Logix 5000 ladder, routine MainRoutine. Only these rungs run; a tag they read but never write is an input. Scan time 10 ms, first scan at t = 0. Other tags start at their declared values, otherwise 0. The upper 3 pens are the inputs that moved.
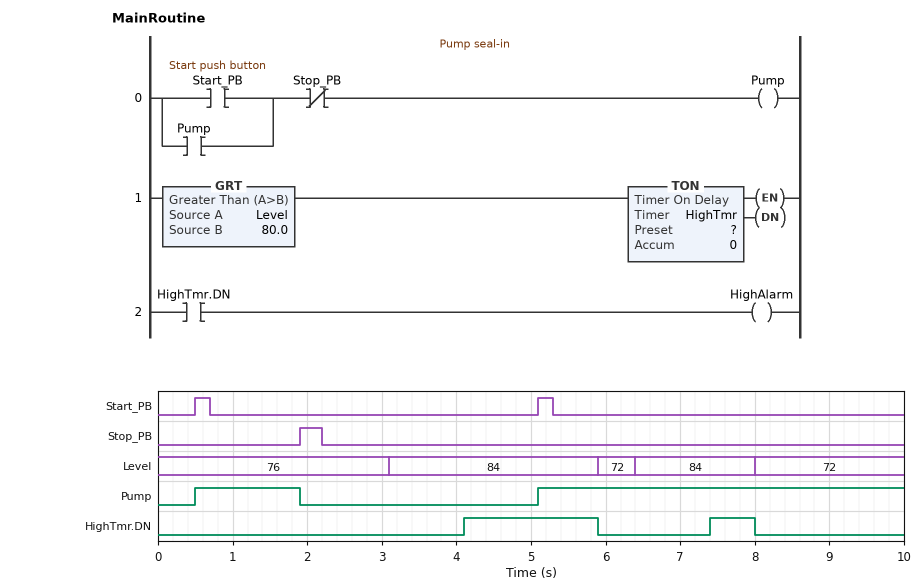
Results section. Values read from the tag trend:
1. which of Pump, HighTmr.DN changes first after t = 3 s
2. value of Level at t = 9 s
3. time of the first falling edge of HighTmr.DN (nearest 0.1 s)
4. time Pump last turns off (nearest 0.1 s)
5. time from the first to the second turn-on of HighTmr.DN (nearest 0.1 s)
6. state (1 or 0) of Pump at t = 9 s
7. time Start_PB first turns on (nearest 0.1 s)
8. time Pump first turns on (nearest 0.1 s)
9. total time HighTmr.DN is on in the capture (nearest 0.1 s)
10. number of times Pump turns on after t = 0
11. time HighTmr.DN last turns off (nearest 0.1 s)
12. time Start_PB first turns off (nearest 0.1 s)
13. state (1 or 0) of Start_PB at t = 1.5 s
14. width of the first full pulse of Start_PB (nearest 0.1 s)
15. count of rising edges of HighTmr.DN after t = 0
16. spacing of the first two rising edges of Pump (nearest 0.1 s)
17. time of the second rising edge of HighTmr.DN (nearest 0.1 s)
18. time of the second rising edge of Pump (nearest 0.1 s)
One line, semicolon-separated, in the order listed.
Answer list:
HighTmr.DN; 72; 5.9 s; 1.9 s; 3.3 s; 1; 0.5 s; 0.5 s; 2.4 s; 2; 8.0 s; 0.7 s; 0; 0.2 s; 2; 4.6 s; 7.4 s; 5.1 s
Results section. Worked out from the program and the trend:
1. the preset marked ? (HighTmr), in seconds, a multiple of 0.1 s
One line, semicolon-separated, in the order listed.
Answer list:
1.0 s
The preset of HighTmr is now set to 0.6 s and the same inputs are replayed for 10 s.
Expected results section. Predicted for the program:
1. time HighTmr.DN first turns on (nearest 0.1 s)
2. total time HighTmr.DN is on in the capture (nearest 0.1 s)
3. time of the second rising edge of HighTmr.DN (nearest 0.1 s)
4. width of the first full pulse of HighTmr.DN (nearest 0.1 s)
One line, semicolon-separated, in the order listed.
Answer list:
3.7 s; 3.2 s; 7.0 s; 2.2 s
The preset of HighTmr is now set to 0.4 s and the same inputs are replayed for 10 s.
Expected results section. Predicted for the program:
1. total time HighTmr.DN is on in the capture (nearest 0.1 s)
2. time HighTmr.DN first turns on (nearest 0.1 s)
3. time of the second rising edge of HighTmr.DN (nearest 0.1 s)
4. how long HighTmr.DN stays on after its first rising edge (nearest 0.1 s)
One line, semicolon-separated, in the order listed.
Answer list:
3.6 s; 3.5 s; 6.8 s; 2.4 s
